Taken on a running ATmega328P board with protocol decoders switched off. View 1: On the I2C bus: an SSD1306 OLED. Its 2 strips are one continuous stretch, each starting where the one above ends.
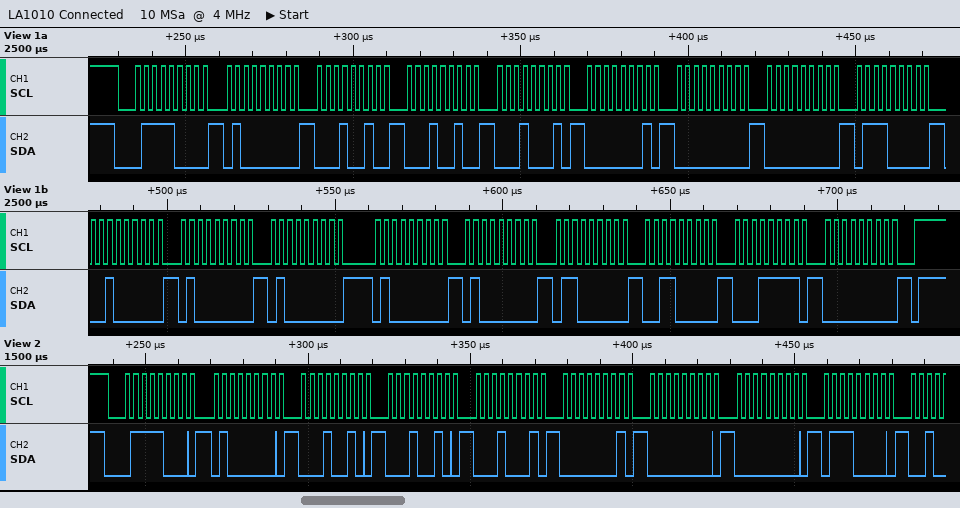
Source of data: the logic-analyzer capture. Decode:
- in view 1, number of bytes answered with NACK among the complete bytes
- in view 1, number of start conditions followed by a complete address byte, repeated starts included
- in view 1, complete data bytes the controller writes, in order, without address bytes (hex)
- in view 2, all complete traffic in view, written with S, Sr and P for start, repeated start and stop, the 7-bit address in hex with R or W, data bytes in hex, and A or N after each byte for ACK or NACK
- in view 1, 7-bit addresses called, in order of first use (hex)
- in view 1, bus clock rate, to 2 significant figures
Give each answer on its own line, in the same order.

0
1
40 12 12 11 01 00 00 70 20 40 40 40 40 60 30 1F 00
S 3CW A 40 A 12 A 12 A 11 A 01 A 00 A 00 A 70 A
0x3C
400 kHz
